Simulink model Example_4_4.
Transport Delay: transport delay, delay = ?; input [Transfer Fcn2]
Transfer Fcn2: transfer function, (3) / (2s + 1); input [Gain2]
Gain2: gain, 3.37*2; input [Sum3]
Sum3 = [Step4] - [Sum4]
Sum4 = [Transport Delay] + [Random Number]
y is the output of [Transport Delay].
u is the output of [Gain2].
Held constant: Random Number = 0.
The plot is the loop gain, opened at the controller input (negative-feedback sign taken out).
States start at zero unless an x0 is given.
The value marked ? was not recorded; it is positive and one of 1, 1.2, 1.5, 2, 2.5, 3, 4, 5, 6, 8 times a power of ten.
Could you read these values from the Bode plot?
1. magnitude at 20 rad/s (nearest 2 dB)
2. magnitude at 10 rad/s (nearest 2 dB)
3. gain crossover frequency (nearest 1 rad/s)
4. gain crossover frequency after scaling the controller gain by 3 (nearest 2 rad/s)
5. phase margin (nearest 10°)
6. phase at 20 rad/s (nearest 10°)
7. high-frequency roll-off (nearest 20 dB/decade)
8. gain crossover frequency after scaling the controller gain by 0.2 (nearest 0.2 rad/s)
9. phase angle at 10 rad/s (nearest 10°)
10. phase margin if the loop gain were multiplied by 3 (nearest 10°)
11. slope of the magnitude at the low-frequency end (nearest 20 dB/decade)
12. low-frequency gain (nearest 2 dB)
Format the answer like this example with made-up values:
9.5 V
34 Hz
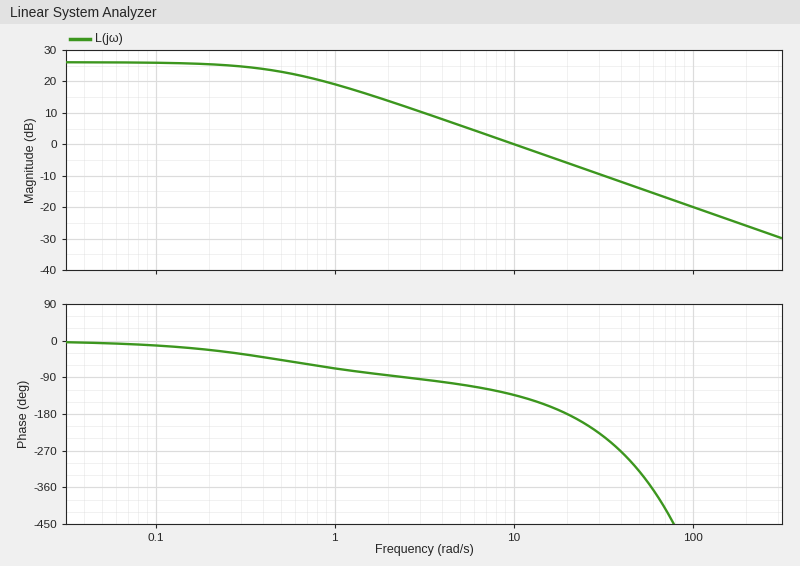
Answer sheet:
-6 dB
0 dB
10 rad/s
30 rad/s
50°
-180°
-20 dB/decade
2.0 rad/s
-130°
-50°
0 dB/decade
26 dB
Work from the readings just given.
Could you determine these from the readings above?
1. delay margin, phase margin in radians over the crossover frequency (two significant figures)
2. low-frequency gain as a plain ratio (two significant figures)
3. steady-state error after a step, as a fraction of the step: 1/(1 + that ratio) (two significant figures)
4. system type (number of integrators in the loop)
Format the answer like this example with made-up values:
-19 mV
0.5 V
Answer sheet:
0.087 s
20
0.048
0
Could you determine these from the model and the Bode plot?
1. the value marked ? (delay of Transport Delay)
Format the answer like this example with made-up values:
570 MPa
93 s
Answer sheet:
0.08
